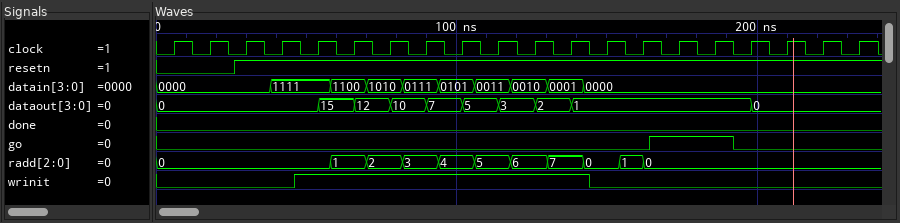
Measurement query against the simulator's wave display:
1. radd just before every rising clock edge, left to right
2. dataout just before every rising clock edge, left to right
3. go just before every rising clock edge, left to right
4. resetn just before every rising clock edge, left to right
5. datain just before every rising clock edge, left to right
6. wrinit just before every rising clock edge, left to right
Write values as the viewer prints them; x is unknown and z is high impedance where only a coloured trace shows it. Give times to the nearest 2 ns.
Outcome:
0, 0, 0, 0, 0, 1, 2, 3, 4, 5, 6, 7, 0, 1, 0, 0, 0, 0, 0, 0
0, 0, 0, 0, 0, 15, 12, 10, 7, 5, 3, 2, 1, 1, 1, 1, 1, 0, 0, 0
0 0 0 0 0 0 0 0 0 0 0 0 0 0 1 1 0 0 0 0
0 0 1 1 1 1 1 1 1 1 1 1 1 1 1 1 1 1 1 1
0000, 0000, 0000, 1111, 1111, 1100, 1010, 0111, 0101, 0011, 0010, 0001, 0000, 0000, 0000, 0000, 0000, 0000, 0000, 0000
0 0 0 0 1 1 1 1 1 1 1 1 0 0 0 0 0 0 0 0
